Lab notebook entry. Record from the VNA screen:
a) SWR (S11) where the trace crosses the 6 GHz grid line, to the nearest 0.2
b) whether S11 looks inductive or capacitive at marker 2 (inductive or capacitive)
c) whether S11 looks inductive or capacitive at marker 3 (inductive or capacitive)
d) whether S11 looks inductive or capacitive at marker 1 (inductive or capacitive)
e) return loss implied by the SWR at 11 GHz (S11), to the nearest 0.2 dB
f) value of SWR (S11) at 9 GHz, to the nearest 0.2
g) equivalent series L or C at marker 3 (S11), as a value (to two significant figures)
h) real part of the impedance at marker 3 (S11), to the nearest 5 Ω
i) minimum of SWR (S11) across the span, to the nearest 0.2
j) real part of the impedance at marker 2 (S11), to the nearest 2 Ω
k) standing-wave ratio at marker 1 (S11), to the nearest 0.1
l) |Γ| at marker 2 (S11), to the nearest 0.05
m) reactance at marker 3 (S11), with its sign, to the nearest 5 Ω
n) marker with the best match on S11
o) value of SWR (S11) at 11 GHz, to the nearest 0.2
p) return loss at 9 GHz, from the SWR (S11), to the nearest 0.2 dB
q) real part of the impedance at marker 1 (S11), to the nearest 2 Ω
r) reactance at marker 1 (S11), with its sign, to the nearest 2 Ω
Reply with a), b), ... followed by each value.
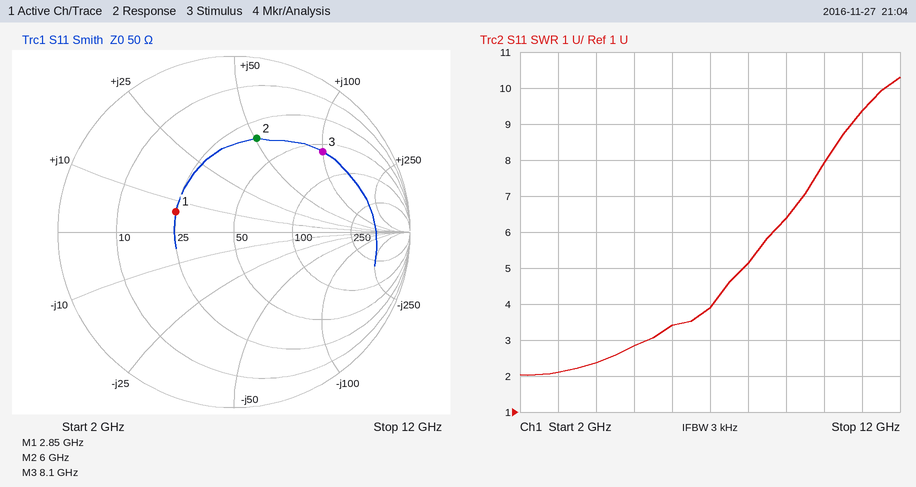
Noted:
a) 3.4
b) inductive
c) inductive
d) inductive
e) 1.8 dB
f) 6.4
g) 2.0 nH
h) 60 Ω
i) 2.0
j) 34 Ω
k) 2.1
l) 0.55
m) +100 Ω
n) marker 1
o) 9.4
p) 2.8 dB
q) 24 Ω
r) +6 Ω
